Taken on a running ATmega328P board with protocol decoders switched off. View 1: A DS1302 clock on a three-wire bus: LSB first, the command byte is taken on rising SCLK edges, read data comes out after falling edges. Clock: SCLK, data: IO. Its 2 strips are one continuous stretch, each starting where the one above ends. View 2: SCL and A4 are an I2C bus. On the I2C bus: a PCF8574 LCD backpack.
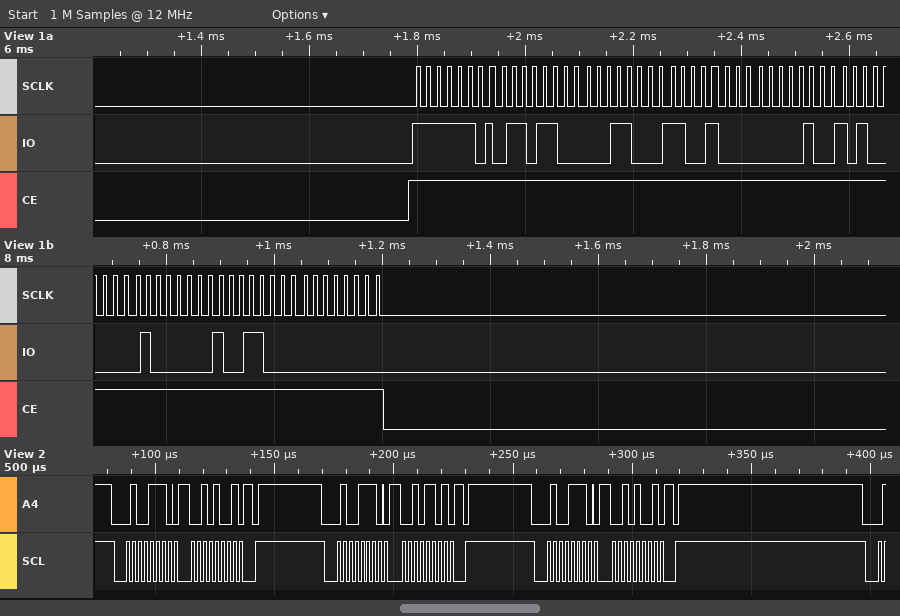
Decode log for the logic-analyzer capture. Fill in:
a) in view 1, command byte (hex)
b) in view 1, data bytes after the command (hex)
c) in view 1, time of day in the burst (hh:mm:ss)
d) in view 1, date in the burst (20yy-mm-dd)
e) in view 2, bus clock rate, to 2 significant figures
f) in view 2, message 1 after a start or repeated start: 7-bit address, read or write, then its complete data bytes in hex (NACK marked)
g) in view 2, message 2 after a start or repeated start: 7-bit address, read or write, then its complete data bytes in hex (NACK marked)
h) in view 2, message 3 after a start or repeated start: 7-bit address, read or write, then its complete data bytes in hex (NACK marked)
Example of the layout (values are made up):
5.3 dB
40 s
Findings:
0xBF
36 18 13 20 05 02 19 00
13:18:36
2019-05-20
400 kHz
0x27 write: 29
0x27 write: 2D
0x27 write: 29
